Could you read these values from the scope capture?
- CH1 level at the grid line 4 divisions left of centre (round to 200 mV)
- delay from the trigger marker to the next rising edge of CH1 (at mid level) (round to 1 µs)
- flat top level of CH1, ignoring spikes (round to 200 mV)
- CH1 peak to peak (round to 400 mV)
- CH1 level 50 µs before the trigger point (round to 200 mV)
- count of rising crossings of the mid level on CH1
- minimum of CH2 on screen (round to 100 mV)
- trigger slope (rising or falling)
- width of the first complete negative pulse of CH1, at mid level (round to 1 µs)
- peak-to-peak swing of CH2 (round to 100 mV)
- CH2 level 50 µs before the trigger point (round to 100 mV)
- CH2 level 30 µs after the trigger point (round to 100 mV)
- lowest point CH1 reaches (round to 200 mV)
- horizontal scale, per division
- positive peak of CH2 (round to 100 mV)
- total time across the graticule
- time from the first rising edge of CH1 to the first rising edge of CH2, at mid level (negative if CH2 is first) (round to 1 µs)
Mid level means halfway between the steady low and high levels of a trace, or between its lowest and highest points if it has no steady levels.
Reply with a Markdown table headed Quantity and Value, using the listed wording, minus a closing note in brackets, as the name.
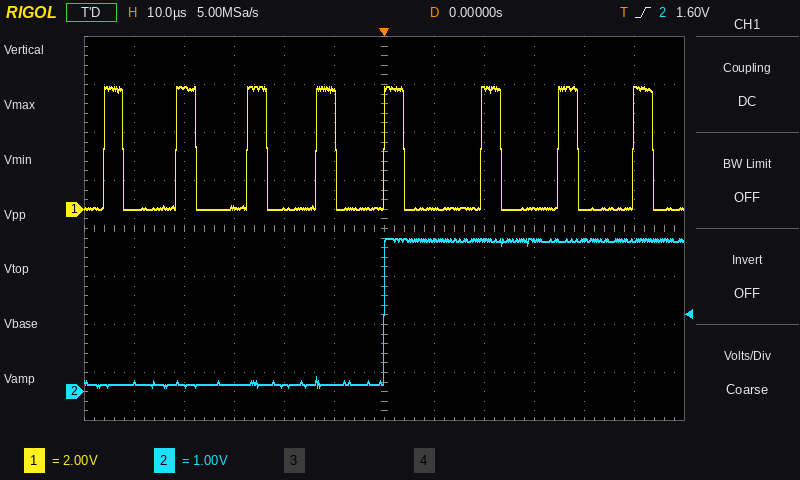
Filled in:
| Quantity | Value |
|---|---|
| CH1 level at the grid line 4 divisions left of centre | 5.0 V |
| delay from the trigger marker to the next rising edge of CH1 (at mid level) | 19 µs |
| flat top level of CH1, ignoring spikes | 5.0 V |
| CH1 peak to peak | 5.2 V |
| CH1 level 50 µs before the trigger point | 0.0 V |
| count of rising crossings of the mid level on CH1 | 8 |
| minimum of CH2 on screen | 100 mV |
| trigger slope | rising |
| width of the first complete negative pulse of CH1, at mid level | 11 µs |
| peak-to-peak swing of CH2 | 3.1 V |
| CH2 level 50 µs before the trigger point | 200 mV |
| CH2 level 30 µs after the trigger point | 3.2 V |
| lowest point CH1 reaches | 0.0 V |
| horizontal scale, per division | 10 µs |
| positive peak of CH2 | 3.2 V |
| total time across the graticule | 120 µs |
| time from the first rising edge of CH1 to the first rising edge of CH2, at mid level (negative if CH2 is first) | +56 µs |
